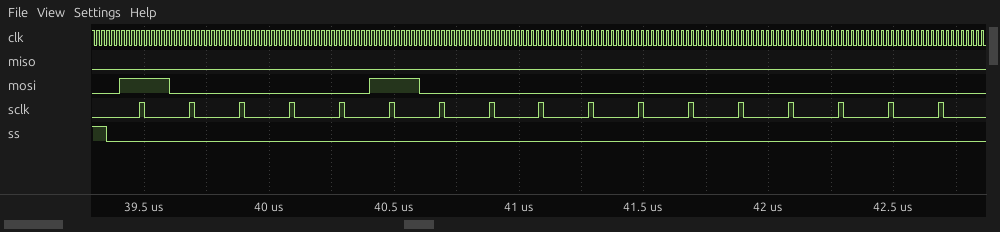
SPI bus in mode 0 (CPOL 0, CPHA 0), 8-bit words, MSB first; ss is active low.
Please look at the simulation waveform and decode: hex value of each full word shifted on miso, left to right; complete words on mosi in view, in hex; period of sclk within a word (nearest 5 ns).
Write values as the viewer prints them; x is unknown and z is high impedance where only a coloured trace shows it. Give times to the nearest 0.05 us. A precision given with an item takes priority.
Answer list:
00, 00
84, 00
200 ns
